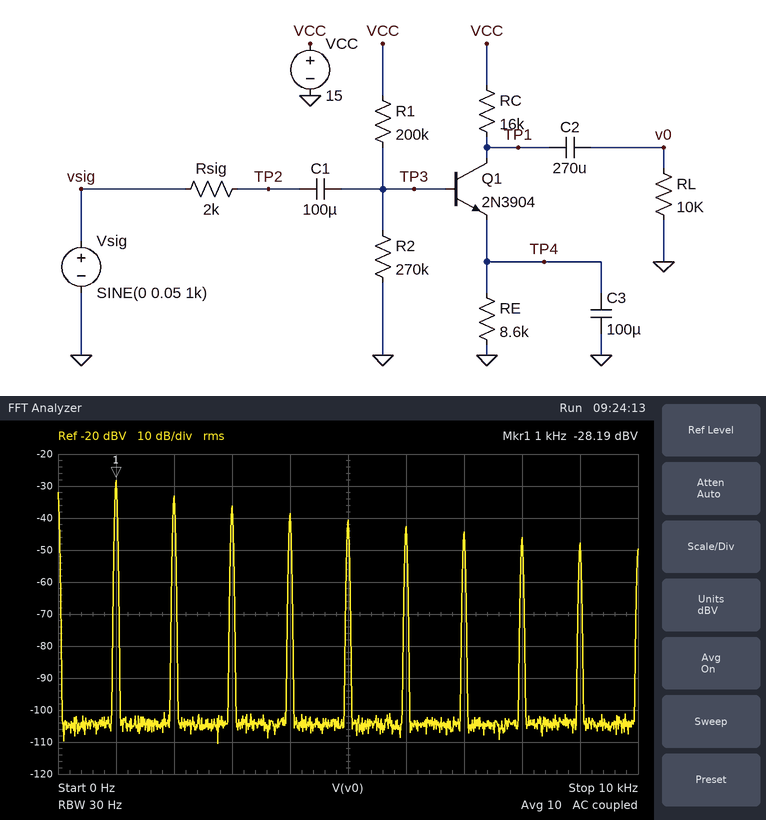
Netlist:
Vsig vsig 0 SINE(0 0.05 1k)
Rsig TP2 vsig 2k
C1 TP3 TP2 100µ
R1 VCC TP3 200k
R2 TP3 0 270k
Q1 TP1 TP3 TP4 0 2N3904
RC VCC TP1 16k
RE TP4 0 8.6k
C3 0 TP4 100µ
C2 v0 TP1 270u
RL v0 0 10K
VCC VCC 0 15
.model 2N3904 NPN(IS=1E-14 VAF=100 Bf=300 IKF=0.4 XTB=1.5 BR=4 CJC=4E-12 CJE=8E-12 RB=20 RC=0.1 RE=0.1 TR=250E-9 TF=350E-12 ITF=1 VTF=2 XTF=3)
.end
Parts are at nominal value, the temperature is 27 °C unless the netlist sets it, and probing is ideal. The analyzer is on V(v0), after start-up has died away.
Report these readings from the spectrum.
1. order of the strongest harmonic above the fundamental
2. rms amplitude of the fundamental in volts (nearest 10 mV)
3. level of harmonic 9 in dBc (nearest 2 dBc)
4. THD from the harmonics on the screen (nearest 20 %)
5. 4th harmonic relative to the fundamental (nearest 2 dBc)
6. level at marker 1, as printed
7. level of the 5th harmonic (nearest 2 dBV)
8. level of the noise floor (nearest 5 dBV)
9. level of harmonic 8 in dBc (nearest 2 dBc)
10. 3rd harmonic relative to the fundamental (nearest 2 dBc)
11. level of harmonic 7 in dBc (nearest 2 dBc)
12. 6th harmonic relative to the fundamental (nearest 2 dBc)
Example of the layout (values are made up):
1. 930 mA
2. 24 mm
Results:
1. 2
2. 40 mV
3. -20 dBc
4. 80 %
5. -10 dBc
6. -28.19 dBV
7. -40 dBV
8. -105 dBV
9. -18 dBc
10. -8 dBc
11. -16 dBc
12. -14 dBc
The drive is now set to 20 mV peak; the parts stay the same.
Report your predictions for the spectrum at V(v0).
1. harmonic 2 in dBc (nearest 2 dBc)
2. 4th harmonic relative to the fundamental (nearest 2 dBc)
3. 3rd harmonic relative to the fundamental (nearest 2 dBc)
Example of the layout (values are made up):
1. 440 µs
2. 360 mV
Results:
1. -18 dBc
2. -50 dBc
3. -34 dBc
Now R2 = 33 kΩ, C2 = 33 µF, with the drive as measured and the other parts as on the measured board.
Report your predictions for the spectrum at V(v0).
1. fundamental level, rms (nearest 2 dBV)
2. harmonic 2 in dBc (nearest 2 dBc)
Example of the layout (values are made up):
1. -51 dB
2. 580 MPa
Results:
1. 0 dBV
2. -8 dBc
